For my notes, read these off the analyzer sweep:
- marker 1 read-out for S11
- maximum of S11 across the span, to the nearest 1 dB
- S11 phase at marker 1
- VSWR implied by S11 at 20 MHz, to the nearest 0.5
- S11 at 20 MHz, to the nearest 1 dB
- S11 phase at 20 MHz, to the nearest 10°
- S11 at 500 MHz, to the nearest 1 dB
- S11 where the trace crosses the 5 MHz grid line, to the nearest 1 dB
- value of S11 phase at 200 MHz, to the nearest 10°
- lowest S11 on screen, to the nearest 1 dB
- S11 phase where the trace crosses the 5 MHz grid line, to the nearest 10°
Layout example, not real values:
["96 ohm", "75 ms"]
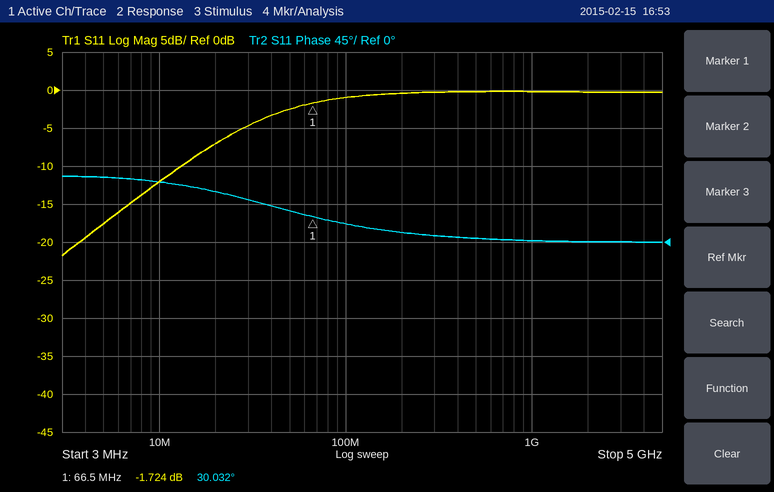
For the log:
["-1.724 dB", "0 dB", "30.032°", "2.5", "-7 dB", "60°", "0 dB", "-18 dB", "10°", "-22 dB", "80°"]
